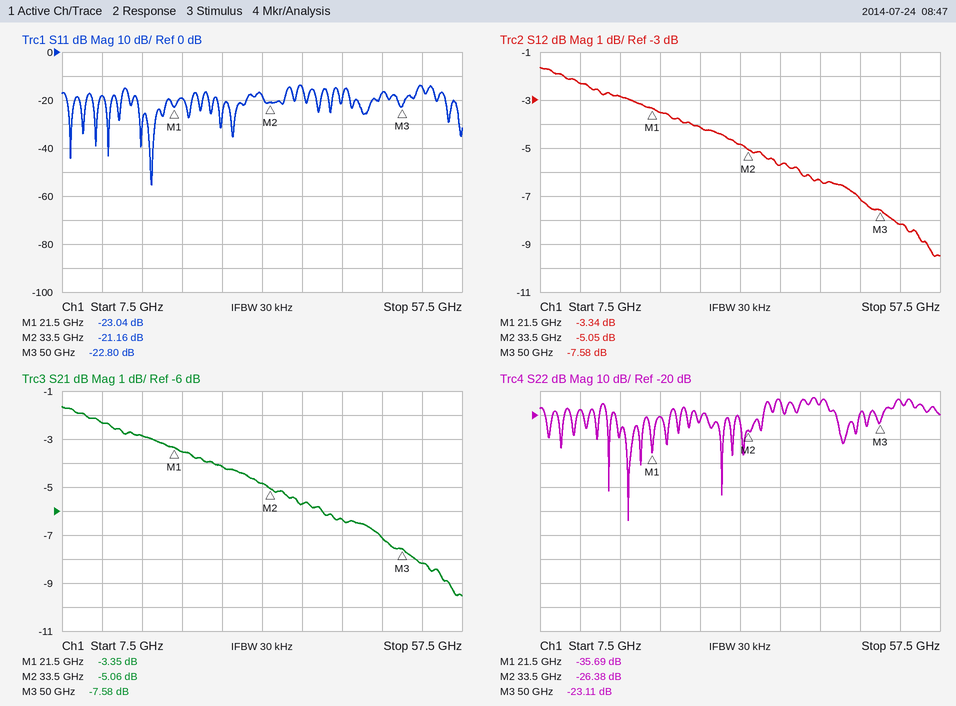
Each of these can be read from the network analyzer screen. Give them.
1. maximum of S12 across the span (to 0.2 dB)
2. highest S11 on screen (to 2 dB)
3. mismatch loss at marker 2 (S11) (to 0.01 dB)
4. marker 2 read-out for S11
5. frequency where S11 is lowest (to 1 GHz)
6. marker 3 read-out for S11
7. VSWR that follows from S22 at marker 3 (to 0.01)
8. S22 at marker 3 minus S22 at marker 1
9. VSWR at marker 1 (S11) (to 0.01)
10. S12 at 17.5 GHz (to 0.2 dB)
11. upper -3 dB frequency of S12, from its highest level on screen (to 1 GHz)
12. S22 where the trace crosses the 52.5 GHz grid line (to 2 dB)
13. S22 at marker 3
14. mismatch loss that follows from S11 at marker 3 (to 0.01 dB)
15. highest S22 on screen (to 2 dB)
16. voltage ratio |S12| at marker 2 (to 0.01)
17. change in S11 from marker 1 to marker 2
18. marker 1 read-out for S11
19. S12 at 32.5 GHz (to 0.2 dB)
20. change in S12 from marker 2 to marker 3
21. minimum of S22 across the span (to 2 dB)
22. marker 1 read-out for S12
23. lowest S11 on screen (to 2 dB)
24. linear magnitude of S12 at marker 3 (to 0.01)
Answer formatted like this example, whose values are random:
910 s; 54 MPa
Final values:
-1.6 dB; -14 dB; 0.03 dB; -21.16 dB; 19 GHz; -22.80 dB; 1.15; 12.58 dB; 1.15; -2.8 dB; 31 GHz; -14 dB; -23.11 dB; 0.02 dB; -12 dB; 0.56; 1.88 dB; -23.04 dB; -4.8 dB; -2.53 dB; -64 dB; -3.34 dB; -56 dB; 0.42
